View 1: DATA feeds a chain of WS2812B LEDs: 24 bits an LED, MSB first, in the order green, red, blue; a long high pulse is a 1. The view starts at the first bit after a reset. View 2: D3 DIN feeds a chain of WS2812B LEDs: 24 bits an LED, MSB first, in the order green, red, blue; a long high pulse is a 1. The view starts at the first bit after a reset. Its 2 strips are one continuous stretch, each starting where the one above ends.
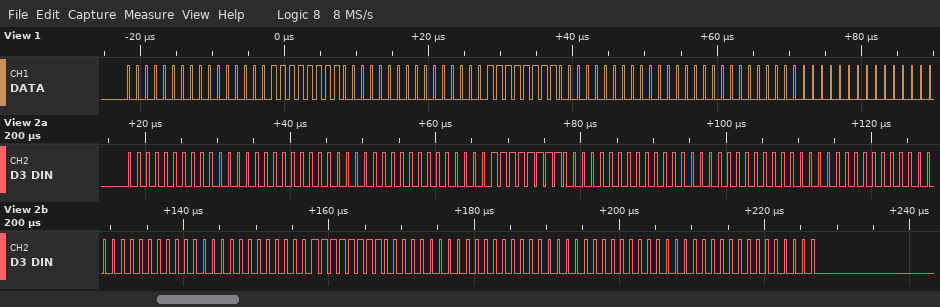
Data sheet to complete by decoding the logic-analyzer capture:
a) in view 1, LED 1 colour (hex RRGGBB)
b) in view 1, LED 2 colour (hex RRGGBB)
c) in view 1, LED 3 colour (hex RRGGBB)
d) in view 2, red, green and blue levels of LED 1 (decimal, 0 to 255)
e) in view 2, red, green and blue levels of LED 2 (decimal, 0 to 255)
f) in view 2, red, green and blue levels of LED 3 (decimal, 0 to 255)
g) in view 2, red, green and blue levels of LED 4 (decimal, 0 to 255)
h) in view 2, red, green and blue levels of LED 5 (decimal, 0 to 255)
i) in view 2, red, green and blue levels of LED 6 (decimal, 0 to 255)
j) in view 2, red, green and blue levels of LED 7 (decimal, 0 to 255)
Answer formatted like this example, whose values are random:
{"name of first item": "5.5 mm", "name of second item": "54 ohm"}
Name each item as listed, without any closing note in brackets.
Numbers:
{"in view 1, LED 1 colour": "#0000FF", "in view 1, LED 2 colour": "#0000FF", "in view 1, LED 3 colour": "#000000", "in view 2, red, green and blue levels of LED 1": "0, 0, 0", "in view 2, red, green and blue levels of LED 2": "0, 0, 255", "in view 2, red, green and blue levels of LED 3": "0, 0, 0", "in view 2, red, green and blue levels of LED 4": "0, 0, 0", "in view 2, red, green and blue levels of LED 5": "0, 0, 255", "in view 2, red, green and blue levels of LED 6": "0, 0, 0", "in view 2, red, green and blue levels of LED 7": "0, 0, 0"}
